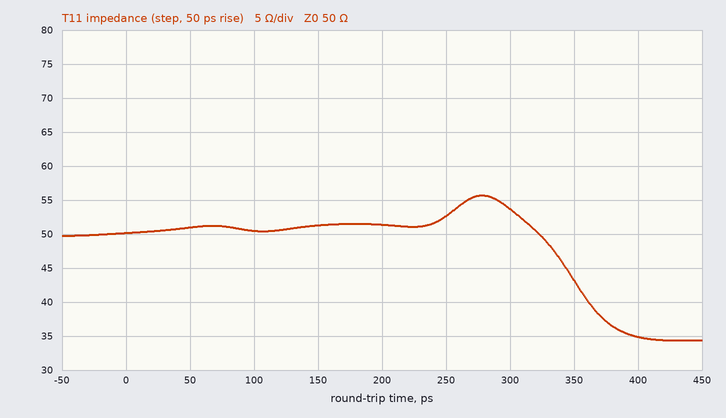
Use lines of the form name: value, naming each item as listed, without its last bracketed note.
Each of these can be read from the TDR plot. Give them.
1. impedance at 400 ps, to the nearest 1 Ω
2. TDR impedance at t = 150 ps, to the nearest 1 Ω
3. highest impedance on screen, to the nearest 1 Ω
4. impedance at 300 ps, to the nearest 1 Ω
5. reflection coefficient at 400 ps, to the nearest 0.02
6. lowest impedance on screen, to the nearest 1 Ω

impedance at 400 ps, to the nearest 1 Ω: 35 Ω
TDR impedance at t = 150 ps, to the nearest 1 Ω: 51 Ω
highest impedance on screen, to the nearest 1 Ω: 56 Ω
impedance at 300 ps, to the nearest 1 Ω: 54 Ω
reflection coefficient at 400 ps, to the nearest 0.02: -0.18
lowest impedance on screen, to the nearest 1 Ω: 34 Ω
